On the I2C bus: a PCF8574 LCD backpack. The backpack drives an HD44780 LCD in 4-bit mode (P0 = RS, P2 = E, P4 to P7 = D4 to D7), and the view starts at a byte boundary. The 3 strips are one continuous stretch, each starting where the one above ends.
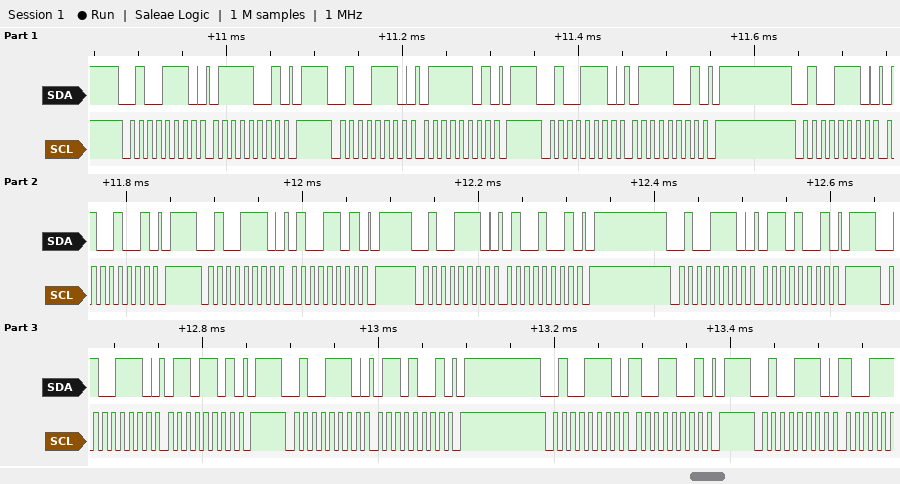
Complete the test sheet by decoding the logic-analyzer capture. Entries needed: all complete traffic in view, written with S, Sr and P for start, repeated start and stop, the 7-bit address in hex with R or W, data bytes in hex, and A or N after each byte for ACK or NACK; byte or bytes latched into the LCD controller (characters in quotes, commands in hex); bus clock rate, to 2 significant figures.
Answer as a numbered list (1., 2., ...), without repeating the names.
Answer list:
1. S 27W A 79 A P S 27W A 7D A P S 27W A 79 A P S 27W A 49 A P S 27W A 4D A P S 27W A 49 A P S 27W A 69 A P S 27W A 6D A P S 27W A 69 A P S 27W A 99 A P S 27W A
2. 't'
3. 100 kHz
